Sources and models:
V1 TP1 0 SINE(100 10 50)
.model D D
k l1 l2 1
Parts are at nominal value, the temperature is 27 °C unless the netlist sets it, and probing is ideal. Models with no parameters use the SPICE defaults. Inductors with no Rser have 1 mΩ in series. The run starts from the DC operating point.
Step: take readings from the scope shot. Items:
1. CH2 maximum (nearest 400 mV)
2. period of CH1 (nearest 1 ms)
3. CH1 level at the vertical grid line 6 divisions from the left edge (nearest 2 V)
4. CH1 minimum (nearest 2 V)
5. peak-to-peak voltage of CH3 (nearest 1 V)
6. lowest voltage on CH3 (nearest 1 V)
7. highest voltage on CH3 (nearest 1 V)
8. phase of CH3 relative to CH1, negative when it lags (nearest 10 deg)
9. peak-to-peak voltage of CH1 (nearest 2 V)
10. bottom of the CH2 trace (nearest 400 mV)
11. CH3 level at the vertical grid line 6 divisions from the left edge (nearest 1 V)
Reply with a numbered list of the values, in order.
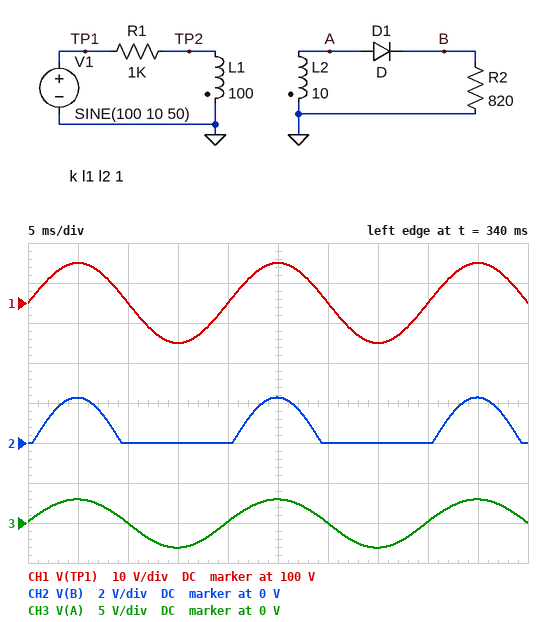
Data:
1. 2.4 V
2. 20 ms
3. 100 V
4. 90 V
5. 6 V
6. -3 V
7. 3 V
8. 0 deg
9. 20 V
10. 0 V
11. 0 V
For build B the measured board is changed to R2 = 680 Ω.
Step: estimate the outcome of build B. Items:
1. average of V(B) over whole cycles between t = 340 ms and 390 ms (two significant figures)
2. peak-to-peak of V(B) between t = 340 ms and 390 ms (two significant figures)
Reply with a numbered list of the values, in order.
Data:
1. 640 mV
2. 2.2 V
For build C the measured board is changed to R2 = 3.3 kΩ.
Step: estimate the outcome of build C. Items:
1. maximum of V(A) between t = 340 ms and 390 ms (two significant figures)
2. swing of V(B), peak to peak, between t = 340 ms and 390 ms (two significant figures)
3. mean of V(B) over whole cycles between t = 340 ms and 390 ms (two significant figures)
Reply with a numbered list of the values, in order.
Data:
1. 3.1 V
2. 2.5 V
3. 700 mV
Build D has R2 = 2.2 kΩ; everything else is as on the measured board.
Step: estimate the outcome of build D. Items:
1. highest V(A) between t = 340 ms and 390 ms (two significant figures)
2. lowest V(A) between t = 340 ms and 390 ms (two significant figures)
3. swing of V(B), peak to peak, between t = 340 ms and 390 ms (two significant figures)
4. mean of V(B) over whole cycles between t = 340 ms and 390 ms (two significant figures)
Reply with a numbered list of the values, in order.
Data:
1. 3.1 V
2. -3.1 V
3. 2.4 V
4. 690 mV
